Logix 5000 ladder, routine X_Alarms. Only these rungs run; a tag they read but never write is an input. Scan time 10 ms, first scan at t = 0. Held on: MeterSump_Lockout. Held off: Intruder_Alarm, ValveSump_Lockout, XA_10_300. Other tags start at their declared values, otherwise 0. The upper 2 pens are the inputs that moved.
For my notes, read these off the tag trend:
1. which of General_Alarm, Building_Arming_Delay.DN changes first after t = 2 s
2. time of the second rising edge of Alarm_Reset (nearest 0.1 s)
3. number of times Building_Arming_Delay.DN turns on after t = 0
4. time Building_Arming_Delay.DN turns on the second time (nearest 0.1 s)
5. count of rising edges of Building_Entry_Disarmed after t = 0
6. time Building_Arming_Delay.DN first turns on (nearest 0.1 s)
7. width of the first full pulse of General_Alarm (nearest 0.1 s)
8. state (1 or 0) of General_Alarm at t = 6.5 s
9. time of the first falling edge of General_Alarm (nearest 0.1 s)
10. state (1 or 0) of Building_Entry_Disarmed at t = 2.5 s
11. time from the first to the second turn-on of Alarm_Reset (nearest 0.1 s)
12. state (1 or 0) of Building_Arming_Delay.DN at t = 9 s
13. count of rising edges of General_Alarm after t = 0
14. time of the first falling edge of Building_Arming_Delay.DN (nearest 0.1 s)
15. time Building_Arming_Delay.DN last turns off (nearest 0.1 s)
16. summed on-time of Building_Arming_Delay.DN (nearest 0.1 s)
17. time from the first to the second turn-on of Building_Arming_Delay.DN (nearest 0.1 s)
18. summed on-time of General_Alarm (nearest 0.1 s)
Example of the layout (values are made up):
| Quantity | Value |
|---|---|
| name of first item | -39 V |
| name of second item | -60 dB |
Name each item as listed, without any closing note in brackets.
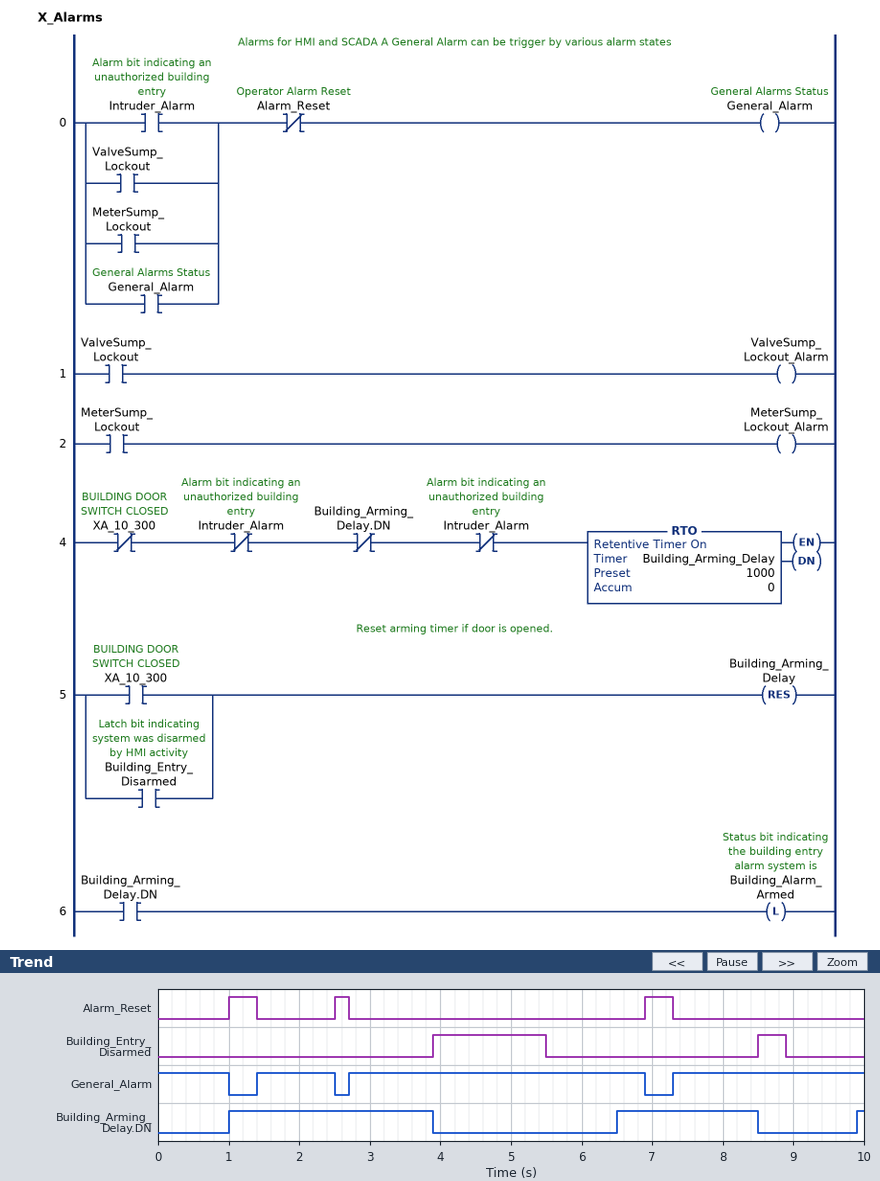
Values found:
| Quantity | Value |
|---|---|
| which of General_Alarm, Building_Arming_Delay.DN changes first after t = 2 s | General_Alarm |
| time of the second rising edge of Alarm_Reset | 2.5 s |
| number of times Building_Arming_Delay.DN turns on after t = 0 | 3 |
| time Building_Arming_Delay.DN turns on the second time | 6.5 s |
| count of rising edges of Building_Entry_Disarmed after t = 0 | 2 |
| time Building_Arming_Delay.DN first turns on | 1.0 s |
| width of the first full pulse of General_Alarm | 1.1 s |
| state (1 or 0) of General_Alarm at t = 6.5 s | 1 |
| time of the first falling edge of General_Alarm | 1.0 s |
| state (1 or 0) of Building_Entry_Disarmed at t = 2.5 s | 0 |
| time from the first to the second turn-on of Alarm_Reset | 1.5 s |
| state (1 or 0) of Building_Arming_Delay.DN at t = 9 s | 0 |
| count of rising edges of General_Alarm after t = 0 | 3 |
| time of the first falling edge of Building_Arming_Delay.DN | 3.9 s |
| time Building_Arming_Delay.DN last turns off | 8.5 s |
| summed on-time of Building_Arming_Delay.DN | 5.0 s |
| time from the first to the second turn-on of Building_Arming_Delay.DN | 5.5 s |
| summed on-time of General_Alarm | 9.0 s |
